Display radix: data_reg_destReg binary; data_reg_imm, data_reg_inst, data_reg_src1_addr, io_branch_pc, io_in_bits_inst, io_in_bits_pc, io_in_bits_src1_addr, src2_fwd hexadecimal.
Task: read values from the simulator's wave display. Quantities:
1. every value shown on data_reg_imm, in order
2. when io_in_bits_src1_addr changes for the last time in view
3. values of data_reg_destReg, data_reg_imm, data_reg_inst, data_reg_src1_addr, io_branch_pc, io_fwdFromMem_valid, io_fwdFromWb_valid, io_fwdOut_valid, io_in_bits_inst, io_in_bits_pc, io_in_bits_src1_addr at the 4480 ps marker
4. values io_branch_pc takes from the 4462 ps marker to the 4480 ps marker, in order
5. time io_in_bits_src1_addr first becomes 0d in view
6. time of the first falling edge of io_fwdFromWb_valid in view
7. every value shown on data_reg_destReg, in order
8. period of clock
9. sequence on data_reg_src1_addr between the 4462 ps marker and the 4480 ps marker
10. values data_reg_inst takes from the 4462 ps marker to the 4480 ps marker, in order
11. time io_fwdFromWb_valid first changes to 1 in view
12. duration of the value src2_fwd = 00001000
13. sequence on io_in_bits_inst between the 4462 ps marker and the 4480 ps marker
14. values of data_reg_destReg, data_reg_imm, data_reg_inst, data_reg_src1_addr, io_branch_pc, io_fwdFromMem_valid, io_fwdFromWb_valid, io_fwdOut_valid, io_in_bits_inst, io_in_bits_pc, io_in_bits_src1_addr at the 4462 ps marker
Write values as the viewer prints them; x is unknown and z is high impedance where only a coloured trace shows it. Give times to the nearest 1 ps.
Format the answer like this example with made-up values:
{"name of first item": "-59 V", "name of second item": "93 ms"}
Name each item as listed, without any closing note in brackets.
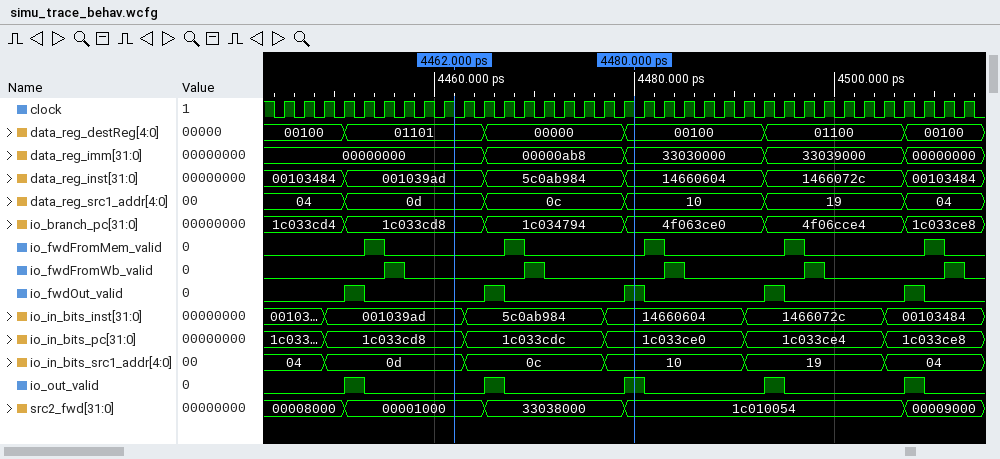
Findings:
{"every value shown on data_reg_imm, in order": "00000000, 00000ab8, 33030000, 33039000, 00000000", "when io_in_bits_src1_addr changes for the last time in view": "4505 ps", "values of data_reg_destReg, data_reg_imm, data_reg_inst, data_reg_src1_addr, io_branch_pc, io_fwdFromMem_valid, io_fwdFromWb_valid, io_fwdOut_valid, io_in_bits_inst, io_in_bits_pc, io_in_bits_src1_addr at the 4480 ps marker": "data_reg_destReg=00100, data_reg_imm=33030000, data_reg_inst=14660604, data_reg_src1_addr=10, io_branch_pc=4f063ce0, io_fwdFromMem_valid=0, io_fwdFromWb_valid=0, io_fwdOut_valid=1, io_in_bits_inst=14660604, io_in_bits_pc=1c033ce0, io_in_bits_src1_addr=10", "values io_branch_pc takes from the 4462 ps marker to the 4480 ps marker, in order": "1c033cd8, 1c034794, 4f063ce0", "time io_in_bits_src1_addr first becomes 0d in view": "4449 ps", "time of the first falling edge of io_fwdFromWb_valid in view": "4457 ps", "every value shown on data_reg_destReg, in order": "00100, 01101, 00000, 00100, 01100, 00100", "period of clock": "2 ps", "sequence on data_reg_src1_addr between the 4462 ps marker and the 4480 ps marker": "0d, 0c, 10", "values data_reg_inst takes from the 4462 ps marker to the 4480 ps marker, in order": "001039ad, 5c0ab984, 14660604", "time io_fwdFromWb_valid first changes to 1 in view": "4455 ps", "duration of the value src2_fwd = 00001000": "14 ps", "sequence on io_in_bits_inst between the 4462 ps marker and the 4480 ps marker": "001039ad, 5c0ab984, 14660604", "values of data_reg_destReg, data_reg_imm, data_reg_inst, data_reg_src1_addr, io_branch_pc, io_fwdFromMem_valid, io_fwdFromWb_valid, io_fwdOut_valid, io_in_bits_inst, io_in_bits_pc, io_in_bits_src1_addr at the 4462 ps marker": "data_reg_destReg=01101, data_reg_imm=00000000, data_reg_inst=001039ad, data_reg_src1_addr=0d, io_branch_pc=1c033cd8, io_fwdFromMem_valid=0, io_fwdFromWb_valid=0, io_fwdOut_valid=0, io_in_bits_inst=001039ad, io_in_bits_pc=1c033cd8, io_in_bits_src1_addr=0d"}
